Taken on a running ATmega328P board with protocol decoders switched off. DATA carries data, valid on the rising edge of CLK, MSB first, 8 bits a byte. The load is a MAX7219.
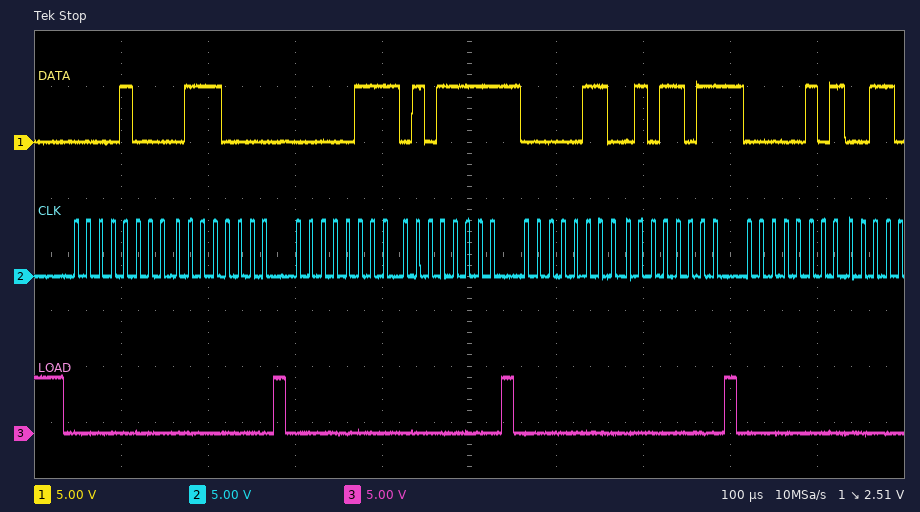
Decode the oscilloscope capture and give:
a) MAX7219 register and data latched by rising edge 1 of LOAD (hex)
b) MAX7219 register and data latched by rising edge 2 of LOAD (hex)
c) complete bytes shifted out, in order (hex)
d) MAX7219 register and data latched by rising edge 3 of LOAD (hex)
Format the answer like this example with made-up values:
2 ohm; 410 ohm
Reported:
register 0x8, data 0x70; register 0x7, data 0x5F; 08 70 07 5F 06 5B 05; register 0x6, data 0x5B
